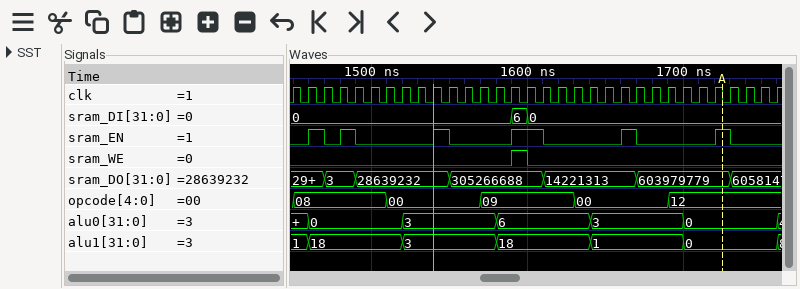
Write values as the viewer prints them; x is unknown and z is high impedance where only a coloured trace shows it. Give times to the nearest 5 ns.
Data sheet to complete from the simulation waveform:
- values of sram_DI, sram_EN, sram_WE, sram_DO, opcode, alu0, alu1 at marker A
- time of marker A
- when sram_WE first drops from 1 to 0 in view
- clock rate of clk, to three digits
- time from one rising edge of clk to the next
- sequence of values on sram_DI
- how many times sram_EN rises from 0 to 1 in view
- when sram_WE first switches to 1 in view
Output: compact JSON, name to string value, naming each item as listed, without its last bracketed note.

{"values of sram_DI, sram_EN, sram_WE, sram_DO, opcode, alu0, alu1 at marker A": "sram_DI=0, sram_EN=1, sram_WE=0, sram_DO=603979779, opcode=12, alu0=0, alu1=0", "time of marker A": "1725 ns", "when sram_WE first drops from 1 to 0 in view": "1600 ns", "clock rate of clk, to three digits": "100 MHz", "time from one rising edge of clk to the next": "10 ns", "sequence of values on sram_DI": "0, 6, 0", "how many times sram_EN rises from 0 to 1 in view": "6", "when sram_WE first switches to 1 in view": "1590 ns"}
